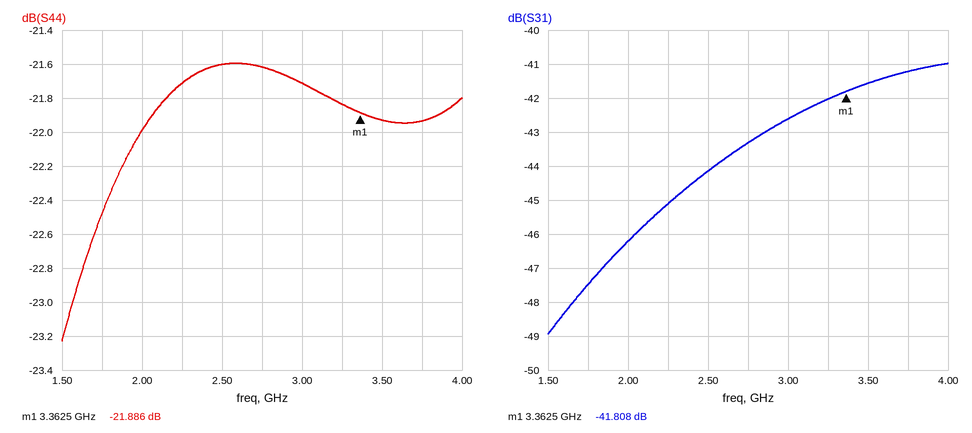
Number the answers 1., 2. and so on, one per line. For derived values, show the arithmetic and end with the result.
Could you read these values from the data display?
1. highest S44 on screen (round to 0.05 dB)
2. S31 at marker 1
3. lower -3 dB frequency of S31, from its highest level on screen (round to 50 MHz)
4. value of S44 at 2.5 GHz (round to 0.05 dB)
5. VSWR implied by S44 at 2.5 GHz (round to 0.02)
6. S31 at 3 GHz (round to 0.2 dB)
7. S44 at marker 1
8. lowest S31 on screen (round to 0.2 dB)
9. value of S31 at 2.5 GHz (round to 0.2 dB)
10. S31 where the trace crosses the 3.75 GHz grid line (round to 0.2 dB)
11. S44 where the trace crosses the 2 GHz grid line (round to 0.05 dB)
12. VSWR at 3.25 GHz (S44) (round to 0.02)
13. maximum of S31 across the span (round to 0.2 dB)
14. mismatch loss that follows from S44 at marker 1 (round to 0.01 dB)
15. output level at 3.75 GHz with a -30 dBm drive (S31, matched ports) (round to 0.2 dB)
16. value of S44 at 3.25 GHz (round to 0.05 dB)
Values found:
1. -21.60 dB
2. -41.808 dB
3. 2.55 GHz
4. -21.60 dB
5. |Γ| = 10^(-21.6/20) = 0.0832; VSWR = (1 + 0.0832)/(1 − 0.0832) ≈ 1.18
6. -42.6 dB
7. -21.886 dB
8. -49.0 dB
9. -44.2 dB
10. -41.2 dB
11. -22.00 dB
12. |Γ| = 10^(-21.85/20) = 0.0808; VSWR = (1 + 0.0808)/(1 − 0.0808) ≈ 1.18
13. -41.0 dB
14. −10 log10(1 − 10^(-21.886/10)) ≈ 0.03 dB
15. -30 dBm + (-41.2 dB) = -71.2 dBm
16. -21.85 dB
